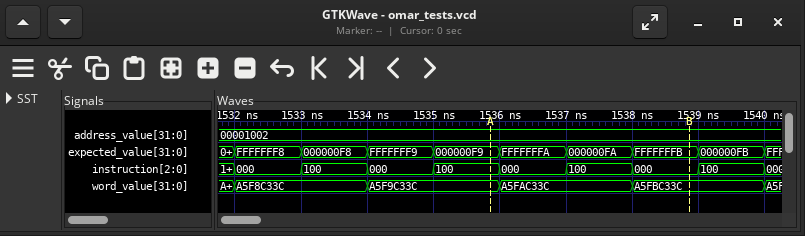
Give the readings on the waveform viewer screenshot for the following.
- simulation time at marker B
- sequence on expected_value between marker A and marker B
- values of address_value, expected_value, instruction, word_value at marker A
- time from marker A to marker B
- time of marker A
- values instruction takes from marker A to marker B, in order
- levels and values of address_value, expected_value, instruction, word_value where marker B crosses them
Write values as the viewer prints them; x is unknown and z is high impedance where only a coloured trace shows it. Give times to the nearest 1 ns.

1539 ns
000000F9, FFFFFFFA, 000000FA, FFFFFFFB
address_value=00001002, expected_value=000000F9, instruction=100, word_value=A5F9C33C
3 ns
1536 ns
100, 000, 100, 000
address_value=00001002, expected_value=FFFFFFFB, instruction=000, word_value=A5FBC33C
